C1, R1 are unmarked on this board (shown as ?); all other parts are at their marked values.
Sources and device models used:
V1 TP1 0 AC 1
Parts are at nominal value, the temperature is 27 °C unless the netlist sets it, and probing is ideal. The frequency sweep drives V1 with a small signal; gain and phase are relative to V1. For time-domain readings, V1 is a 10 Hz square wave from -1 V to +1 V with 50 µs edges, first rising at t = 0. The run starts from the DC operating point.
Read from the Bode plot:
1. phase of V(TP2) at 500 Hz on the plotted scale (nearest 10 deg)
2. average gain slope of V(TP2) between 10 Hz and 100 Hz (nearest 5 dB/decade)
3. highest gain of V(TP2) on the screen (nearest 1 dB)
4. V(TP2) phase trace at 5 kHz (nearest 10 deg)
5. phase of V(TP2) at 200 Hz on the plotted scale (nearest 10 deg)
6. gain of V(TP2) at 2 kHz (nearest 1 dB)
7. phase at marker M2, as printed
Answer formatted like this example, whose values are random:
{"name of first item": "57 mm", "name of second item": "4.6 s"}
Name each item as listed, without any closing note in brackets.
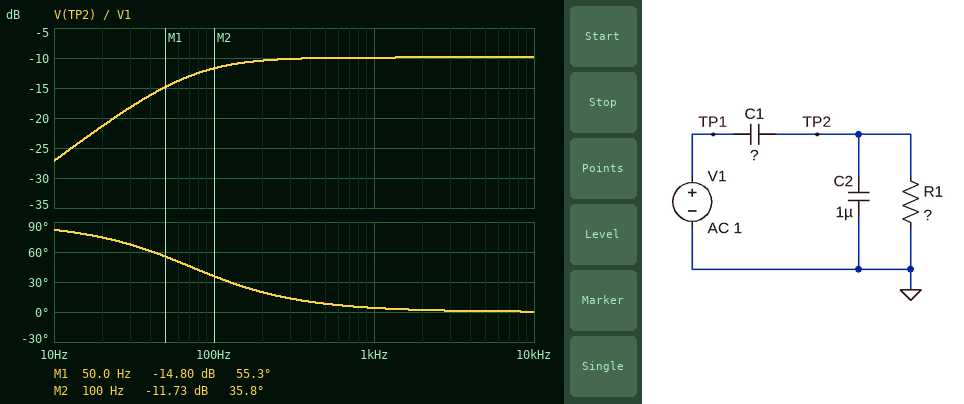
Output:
{"phase of V(TP2) at 500 Hz on the plotted scale": "10 deg", "average gain slope of V(TP2) between 10 Hz and 100 Hz": "15 dB/decade", "highest gain of V(TP2) on the screen": "-10 dB", "V(TP2) phase trace at 5 kHz": "0 deg", "phase of V(TP2) at 200 Hz on the plotted scale": "20 deg", "gain of V(TP2) at 2 kHz": "-10 dB", "phase at marker M2, as printed": "35.8 deg"}
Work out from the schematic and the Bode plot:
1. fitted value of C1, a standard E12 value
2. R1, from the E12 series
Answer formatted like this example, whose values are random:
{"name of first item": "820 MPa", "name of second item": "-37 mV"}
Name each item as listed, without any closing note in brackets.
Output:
{"fitted value of C1, a standard E12 value": "470 nF", "R1, from the E12 series": "1.5 kΩ"}
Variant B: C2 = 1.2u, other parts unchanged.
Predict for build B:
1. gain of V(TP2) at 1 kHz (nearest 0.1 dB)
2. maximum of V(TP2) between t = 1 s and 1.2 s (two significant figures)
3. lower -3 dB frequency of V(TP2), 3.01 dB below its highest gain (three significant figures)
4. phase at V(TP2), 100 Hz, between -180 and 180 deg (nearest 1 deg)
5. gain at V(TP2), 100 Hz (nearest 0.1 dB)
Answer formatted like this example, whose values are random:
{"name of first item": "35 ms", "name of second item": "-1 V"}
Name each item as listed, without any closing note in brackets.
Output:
{"gain of V(TP2) at 1 kHz": "-11.0 dB", "maximum of V(TP2) between t = 1 s and 1.2 s": "560 mV", "lower -3 dB frequency of V(TP2), 3.01 dB below its highest gain": "63.5 Hz", "phase at V(TP2), 100 Hz, between -180 and 180 deg": "32 deg", "gain at V(TP2), 100 Hz": "-12.5 dB"}
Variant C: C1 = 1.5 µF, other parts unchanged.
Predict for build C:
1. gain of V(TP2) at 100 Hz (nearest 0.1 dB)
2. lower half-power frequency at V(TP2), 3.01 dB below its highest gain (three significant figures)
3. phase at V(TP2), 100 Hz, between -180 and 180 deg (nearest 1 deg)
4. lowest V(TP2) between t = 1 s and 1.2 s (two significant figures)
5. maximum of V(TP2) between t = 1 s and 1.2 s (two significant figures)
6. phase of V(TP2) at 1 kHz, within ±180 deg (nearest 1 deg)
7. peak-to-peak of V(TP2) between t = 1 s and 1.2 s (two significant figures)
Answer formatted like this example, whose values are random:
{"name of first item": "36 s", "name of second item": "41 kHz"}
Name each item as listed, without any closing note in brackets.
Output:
{"gain of V(TP2) at 100 Hz": "-5.2 dB", "lower half-power frequency at V(TP2), 3.01 dB below its highest gain": "42.4 Hz", "phase at V(TP2), 100 Hz, between -180 and 180 deg": "23 deg", "lowest V(TP2) between t = 1 s and 1.2 s": "-1.2 V", "maximum of V(TP2) between t = 1 s and 1.2 s": "1.2 V", "phase of V(TP2) at 1 kHz, within ±180 deg": "2 deg", "peak-to-peak of V(TP2) between t = 1 s and 1.2 s": "2.4 V"}
